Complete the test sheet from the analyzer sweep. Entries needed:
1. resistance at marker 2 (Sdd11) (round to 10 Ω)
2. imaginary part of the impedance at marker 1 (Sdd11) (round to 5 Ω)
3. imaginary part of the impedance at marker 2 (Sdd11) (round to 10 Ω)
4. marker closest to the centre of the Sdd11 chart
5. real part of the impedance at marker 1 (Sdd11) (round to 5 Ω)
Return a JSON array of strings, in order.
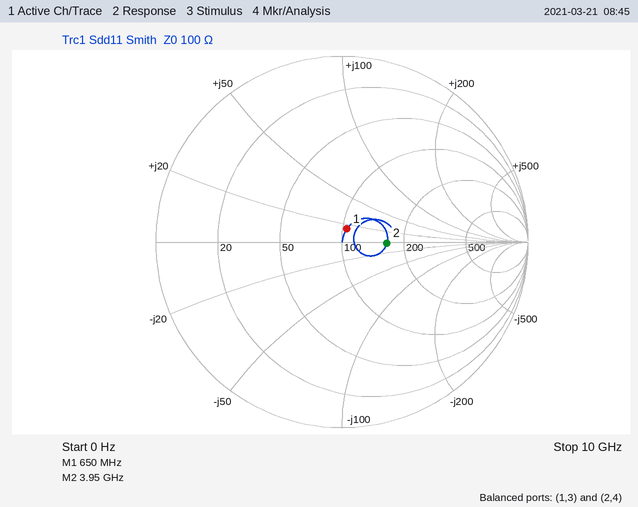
["160 Ω", "+15 Ω", "0 Ω", "marker 1", "105 Ω"]
